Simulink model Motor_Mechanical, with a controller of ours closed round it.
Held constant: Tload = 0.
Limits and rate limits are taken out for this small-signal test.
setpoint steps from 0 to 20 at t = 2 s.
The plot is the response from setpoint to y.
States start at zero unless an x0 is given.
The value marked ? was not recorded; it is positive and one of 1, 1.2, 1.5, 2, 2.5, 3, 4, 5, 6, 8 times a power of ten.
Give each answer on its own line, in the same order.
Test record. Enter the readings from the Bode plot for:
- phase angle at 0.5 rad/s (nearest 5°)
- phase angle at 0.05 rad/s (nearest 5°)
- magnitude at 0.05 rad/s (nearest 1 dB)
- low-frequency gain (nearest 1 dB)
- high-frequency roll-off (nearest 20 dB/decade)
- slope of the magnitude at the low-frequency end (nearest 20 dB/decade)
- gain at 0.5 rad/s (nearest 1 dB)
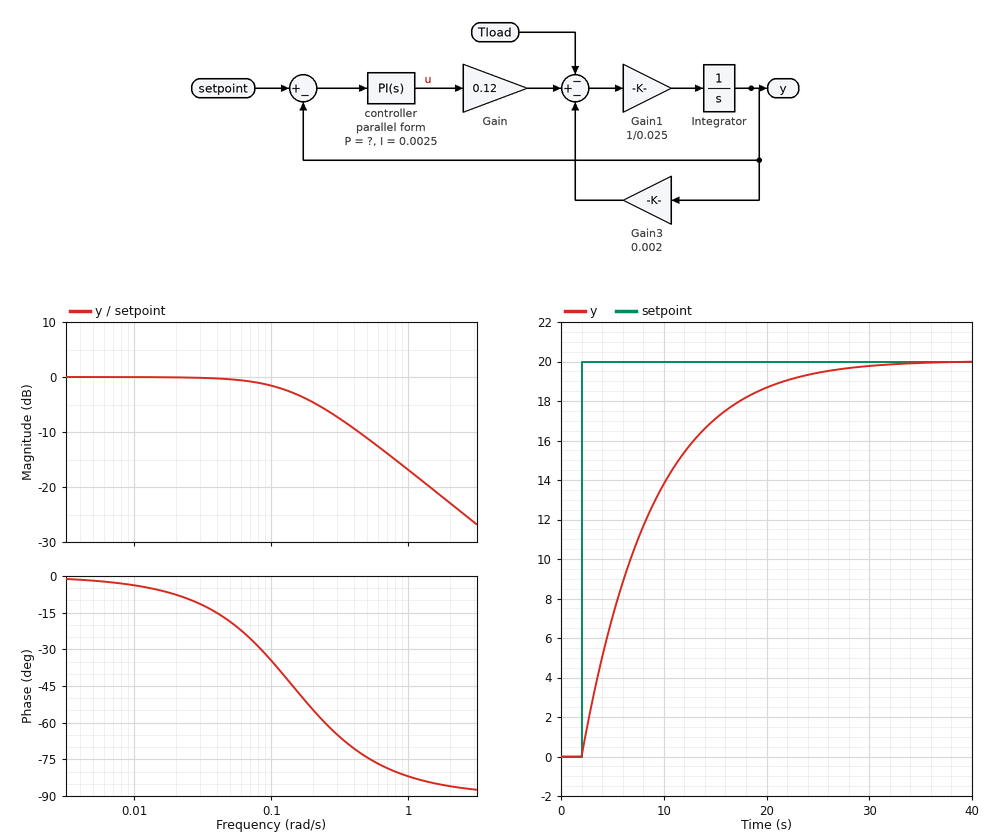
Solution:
-75°
-20°
0 dB
0 dB
-20 dB/decade
0 dB/decade
-11 dB
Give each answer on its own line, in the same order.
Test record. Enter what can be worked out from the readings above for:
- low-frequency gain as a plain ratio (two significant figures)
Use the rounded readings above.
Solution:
1.0
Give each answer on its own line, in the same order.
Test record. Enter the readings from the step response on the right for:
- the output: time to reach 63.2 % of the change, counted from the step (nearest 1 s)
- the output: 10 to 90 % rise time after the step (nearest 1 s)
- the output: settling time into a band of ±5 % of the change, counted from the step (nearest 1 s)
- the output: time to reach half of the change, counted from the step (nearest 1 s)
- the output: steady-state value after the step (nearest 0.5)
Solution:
7 s
15 s
20 s
5 s
20.0
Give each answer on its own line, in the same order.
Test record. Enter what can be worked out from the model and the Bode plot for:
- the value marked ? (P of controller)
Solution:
0.03
